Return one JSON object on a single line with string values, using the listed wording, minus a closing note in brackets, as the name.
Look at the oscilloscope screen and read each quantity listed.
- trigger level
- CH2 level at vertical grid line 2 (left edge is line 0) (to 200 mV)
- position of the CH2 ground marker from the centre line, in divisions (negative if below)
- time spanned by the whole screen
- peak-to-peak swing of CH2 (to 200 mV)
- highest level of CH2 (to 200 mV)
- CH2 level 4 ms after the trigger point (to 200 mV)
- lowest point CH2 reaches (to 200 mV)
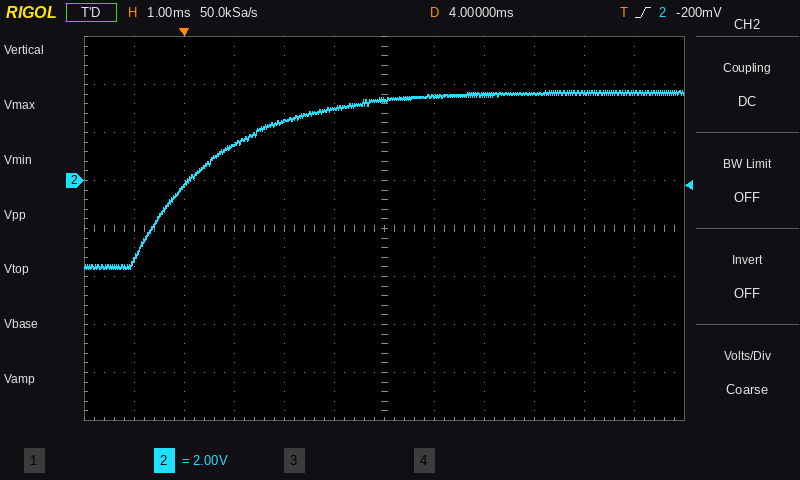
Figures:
{"trigger level": "-200 mV", "CH2 level at vertical grid line 2 (left edge is line 0)": "-200 mV", "position of the CH2 ground marker from the centre line, in divisions": "+1.0 div", "time spanned by the whole screen": "12 ms", "peak-to-peak swing of CH2": "7.4 V", "highest level of CH2": "3.8 V", "CH2 level 4 ms after the trigger point": "3.4 V", "lowest point CH2 reaches": "-3.6 V"}
